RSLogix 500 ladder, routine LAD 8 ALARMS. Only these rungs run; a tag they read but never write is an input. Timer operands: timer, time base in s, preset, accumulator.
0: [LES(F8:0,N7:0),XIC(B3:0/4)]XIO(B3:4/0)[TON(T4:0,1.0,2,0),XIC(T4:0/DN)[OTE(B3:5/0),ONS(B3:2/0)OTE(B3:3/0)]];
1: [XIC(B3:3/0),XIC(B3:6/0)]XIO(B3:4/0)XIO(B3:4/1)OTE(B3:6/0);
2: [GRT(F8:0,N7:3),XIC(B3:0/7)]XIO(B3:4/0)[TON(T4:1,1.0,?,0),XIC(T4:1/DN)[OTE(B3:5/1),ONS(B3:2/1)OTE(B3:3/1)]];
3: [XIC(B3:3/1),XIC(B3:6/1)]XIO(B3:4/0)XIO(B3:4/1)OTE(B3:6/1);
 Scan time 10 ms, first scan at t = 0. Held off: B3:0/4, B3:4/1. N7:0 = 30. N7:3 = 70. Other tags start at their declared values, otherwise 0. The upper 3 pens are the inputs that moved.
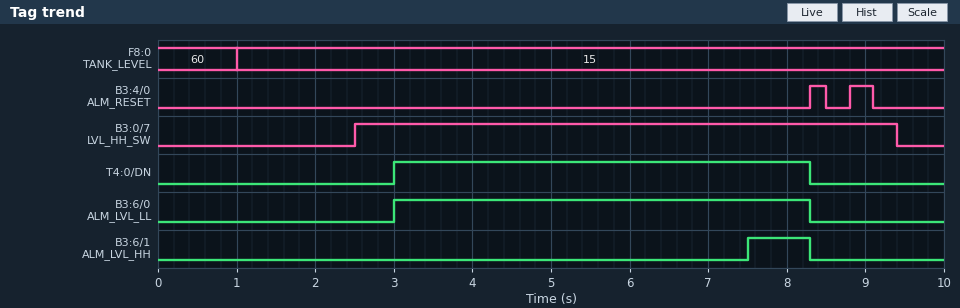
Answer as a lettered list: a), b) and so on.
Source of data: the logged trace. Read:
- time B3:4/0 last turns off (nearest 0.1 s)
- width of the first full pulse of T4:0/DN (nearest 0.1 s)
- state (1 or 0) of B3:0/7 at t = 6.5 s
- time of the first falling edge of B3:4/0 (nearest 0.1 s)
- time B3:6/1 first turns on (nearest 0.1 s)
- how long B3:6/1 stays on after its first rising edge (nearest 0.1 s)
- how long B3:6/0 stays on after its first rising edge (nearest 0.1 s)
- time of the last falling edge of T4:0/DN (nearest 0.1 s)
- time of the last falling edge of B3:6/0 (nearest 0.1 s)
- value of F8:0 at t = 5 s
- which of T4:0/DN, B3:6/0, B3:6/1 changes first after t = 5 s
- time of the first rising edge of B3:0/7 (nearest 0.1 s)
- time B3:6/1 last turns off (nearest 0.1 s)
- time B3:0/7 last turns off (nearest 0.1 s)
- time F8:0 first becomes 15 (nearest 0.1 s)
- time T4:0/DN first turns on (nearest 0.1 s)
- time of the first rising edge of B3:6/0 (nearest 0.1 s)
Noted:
a) 9.1 s
b) 5.3 s
c) 1
d) 8.5 s
e) 7.5 s
f) 0.8 s
g) 5.3 s
h) 8.3 s
i) 8.3 s
j) 15
k) B3:6/1
l) 2.5 s
m) 8.3 s
n) 9.4 s
o) 1.0 s
p) 3.0 s
q) 3.0 s
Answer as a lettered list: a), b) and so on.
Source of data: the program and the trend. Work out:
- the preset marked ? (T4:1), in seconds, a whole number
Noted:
a) 5 s
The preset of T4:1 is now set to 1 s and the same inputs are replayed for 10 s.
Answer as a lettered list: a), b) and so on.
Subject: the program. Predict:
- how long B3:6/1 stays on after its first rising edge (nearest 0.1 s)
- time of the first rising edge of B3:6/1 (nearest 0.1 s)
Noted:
a) 4.8 s
b) 3.5 s
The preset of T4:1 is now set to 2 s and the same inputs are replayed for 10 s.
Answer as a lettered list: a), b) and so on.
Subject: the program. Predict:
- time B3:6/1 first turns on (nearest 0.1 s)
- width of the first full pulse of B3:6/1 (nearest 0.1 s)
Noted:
a) 4.5 s
b) 3.8 s
